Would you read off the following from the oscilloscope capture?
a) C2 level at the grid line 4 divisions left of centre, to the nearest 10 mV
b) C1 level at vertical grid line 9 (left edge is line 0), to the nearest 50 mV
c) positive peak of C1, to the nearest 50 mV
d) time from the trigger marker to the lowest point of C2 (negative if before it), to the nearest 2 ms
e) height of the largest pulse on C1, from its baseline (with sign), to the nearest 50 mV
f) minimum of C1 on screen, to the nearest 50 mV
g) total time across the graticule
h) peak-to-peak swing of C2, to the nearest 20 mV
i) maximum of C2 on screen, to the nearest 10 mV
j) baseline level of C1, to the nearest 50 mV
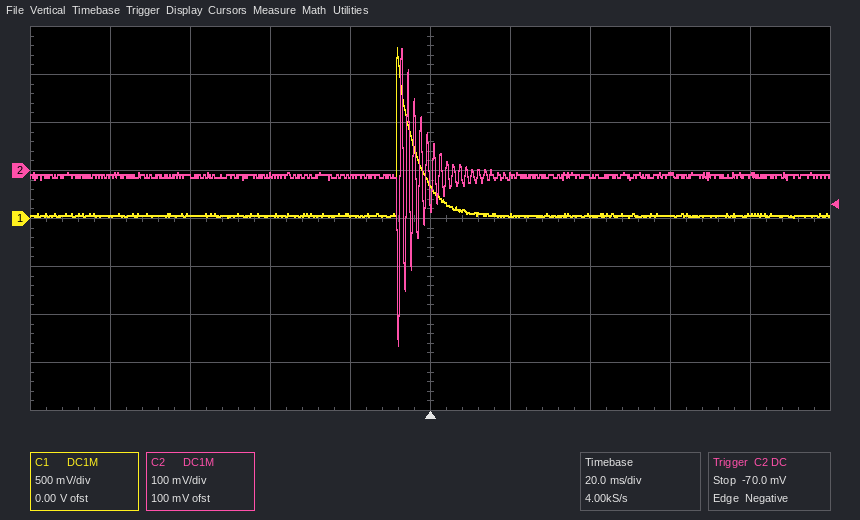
-10 mV
50 mV
1.80 V
-8 ms
+1.75 V
0 mV
200 ms
620 mV
250 mV
50 mV
